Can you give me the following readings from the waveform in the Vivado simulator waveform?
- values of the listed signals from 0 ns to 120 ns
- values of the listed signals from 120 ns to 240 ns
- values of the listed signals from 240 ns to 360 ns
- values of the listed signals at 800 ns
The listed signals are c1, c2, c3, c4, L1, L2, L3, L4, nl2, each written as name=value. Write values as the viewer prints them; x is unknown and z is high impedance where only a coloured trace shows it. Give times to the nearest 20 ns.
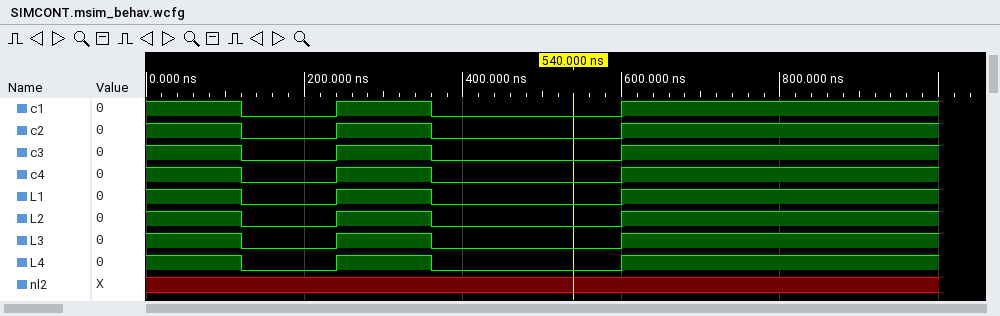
c1=1, c2=1, c3=1, c4=1, L1=1, L2=1, L3=1, L4=1, nl2=x
c1=0, c2=0, c3=0, c4=0, L1=0, L2=0, L3=0, L4=0, nl2=x
c1=1, c2=1, c3=1, c4=1, L1=1, L2=1, L3=1, L4=1, nl2=x
c1=1, c2=1, c3=1, c4=1, L1=1, L2=1, L3=1, L4=1, nl2=x
